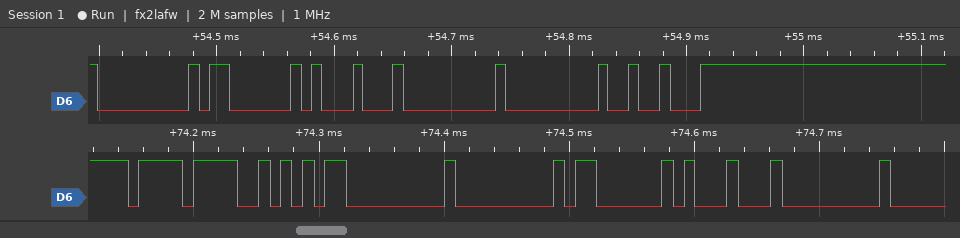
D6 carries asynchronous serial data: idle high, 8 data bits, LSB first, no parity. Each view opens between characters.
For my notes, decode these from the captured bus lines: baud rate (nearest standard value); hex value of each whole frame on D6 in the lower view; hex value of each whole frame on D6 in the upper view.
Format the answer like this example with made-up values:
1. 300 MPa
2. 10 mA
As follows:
1. 115200 baud
2. EF, AA, 00, 00, 03, 11, 00
3. 00, 03, 11, 00, 00, 12
